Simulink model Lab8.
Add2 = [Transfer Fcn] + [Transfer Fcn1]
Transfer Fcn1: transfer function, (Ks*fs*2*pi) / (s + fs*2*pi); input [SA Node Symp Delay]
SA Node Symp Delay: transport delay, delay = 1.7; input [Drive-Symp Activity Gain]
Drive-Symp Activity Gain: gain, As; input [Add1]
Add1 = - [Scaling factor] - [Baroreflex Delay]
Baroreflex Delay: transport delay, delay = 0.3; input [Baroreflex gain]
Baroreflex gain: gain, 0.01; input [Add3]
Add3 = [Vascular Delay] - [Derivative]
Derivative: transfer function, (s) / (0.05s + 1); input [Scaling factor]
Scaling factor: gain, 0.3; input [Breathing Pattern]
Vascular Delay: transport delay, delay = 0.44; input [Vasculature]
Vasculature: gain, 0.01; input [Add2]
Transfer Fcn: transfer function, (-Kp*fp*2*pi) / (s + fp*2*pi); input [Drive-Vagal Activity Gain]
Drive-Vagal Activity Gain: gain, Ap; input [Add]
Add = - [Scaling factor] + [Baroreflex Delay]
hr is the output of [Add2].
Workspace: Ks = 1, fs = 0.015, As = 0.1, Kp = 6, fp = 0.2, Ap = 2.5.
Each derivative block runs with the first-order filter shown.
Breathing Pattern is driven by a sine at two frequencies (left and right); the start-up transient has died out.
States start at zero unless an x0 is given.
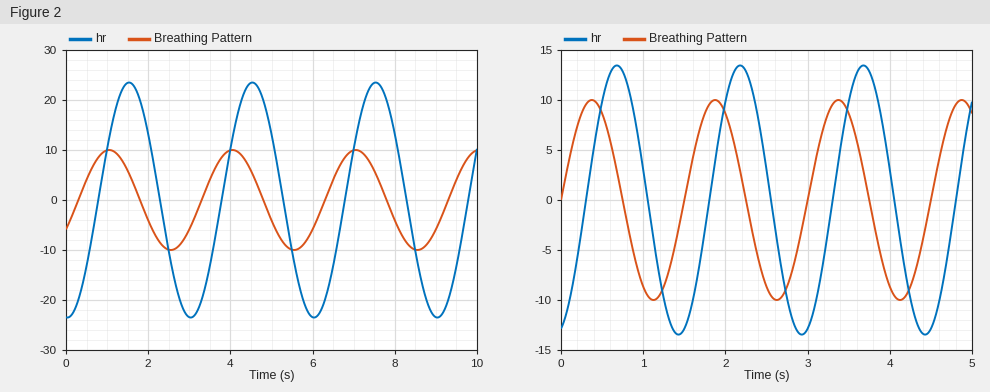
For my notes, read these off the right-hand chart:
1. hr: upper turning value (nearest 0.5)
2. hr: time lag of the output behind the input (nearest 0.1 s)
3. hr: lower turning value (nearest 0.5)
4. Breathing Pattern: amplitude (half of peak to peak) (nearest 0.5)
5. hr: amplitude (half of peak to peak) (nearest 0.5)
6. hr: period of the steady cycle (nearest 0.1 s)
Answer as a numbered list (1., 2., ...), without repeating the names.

1. 13.5
2. 0.3 s
3. -13.5
4. 10.0
5. 13.5
6. 1.5 s
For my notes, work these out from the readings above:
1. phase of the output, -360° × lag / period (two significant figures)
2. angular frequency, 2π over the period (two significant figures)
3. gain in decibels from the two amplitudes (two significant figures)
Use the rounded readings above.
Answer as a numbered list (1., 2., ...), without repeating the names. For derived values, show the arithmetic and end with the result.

1. -360 × 0.3 / 1.5 = -72°
2. 2π / 1.5 = 4.2 rad/s
3. 20 log10(13.5 / 10) = 2.6 dB
